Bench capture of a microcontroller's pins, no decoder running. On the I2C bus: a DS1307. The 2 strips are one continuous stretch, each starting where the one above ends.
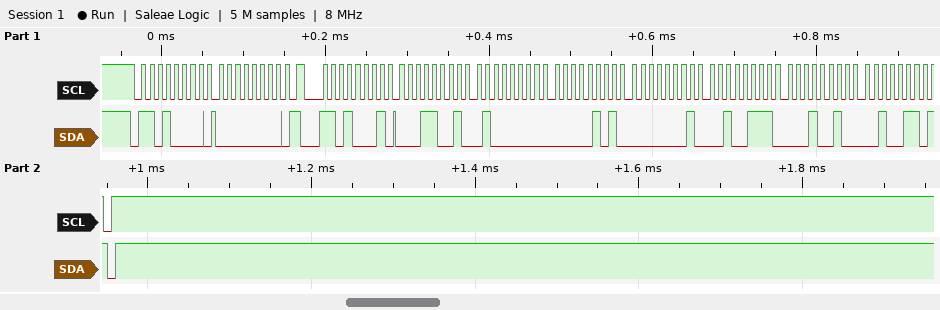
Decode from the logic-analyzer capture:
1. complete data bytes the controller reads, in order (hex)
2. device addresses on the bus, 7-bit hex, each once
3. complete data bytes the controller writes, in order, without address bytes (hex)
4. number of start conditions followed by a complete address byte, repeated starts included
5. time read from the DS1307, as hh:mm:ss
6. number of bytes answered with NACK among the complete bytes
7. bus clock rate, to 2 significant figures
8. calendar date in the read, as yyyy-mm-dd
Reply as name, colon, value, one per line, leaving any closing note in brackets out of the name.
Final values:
complete data bytes the controller reads, in order: 19 40 05 01 27 12 26
device addresses on the bus, 7-bit hex, each once: 0x68
complete data bytes the controller writes, in order, without address bytes: 00
number of start conditions followed by a complete address byte, repeated starts included: 2
time read from the DS1307, as hh:mm:ss: 05:40:19
number of bytes answered with NACK among the complete bytes: 1
bus clock rate, to 2 significant figures: 100 kHz
calendar date in the read, as yyyy-mm-dd: 2026-12-27
